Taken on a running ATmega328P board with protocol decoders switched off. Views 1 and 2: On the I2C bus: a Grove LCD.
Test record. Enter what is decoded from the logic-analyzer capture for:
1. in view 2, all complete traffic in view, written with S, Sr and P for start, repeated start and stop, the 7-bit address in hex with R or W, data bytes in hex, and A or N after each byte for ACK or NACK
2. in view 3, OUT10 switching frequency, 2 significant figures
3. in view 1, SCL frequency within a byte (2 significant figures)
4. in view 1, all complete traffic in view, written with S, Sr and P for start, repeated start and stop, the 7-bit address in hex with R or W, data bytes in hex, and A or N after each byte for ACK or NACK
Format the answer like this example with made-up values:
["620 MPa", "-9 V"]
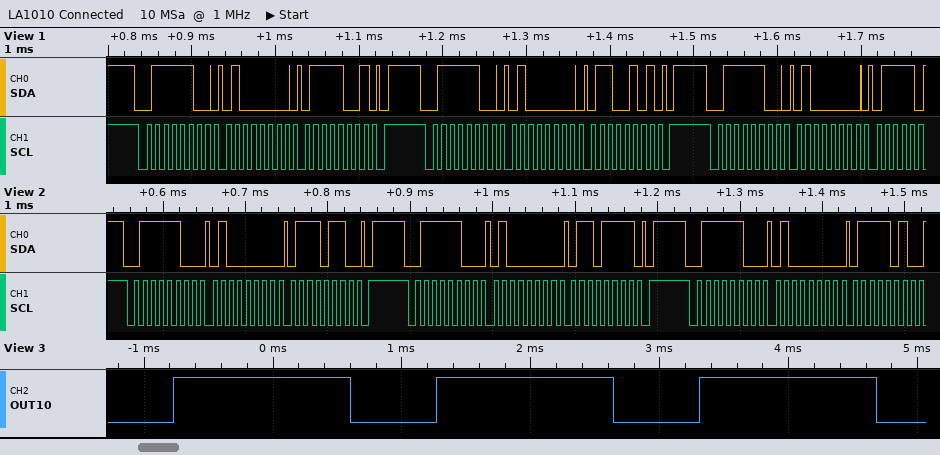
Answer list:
["S 3EW A 40 A 76 A P S 3EW A 40 A 6F A P S 3EW A 40 A 7A A", "490 Hz", "100 kHz", "S 3EW A 40 A 79 A P S 3EW A 40 A 65 A P S 3EW A 40 A"]
